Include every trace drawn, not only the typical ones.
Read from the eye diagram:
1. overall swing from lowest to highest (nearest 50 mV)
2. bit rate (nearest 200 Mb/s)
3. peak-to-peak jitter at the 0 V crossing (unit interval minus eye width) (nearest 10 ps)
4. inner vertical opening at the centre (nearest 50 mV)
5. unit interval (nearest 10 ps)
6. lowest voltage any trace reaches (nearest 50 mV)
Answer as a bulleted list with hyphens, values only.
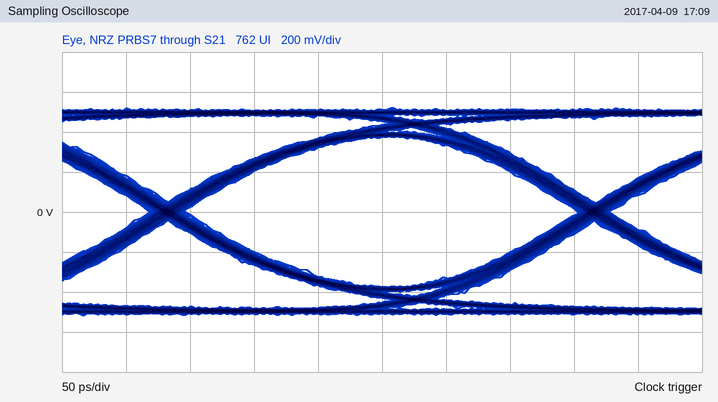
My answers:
- 1.05 V
- 3.0 Gb/s
- 30 ps
- 750 mV
- 330 ps
- -500 mV
